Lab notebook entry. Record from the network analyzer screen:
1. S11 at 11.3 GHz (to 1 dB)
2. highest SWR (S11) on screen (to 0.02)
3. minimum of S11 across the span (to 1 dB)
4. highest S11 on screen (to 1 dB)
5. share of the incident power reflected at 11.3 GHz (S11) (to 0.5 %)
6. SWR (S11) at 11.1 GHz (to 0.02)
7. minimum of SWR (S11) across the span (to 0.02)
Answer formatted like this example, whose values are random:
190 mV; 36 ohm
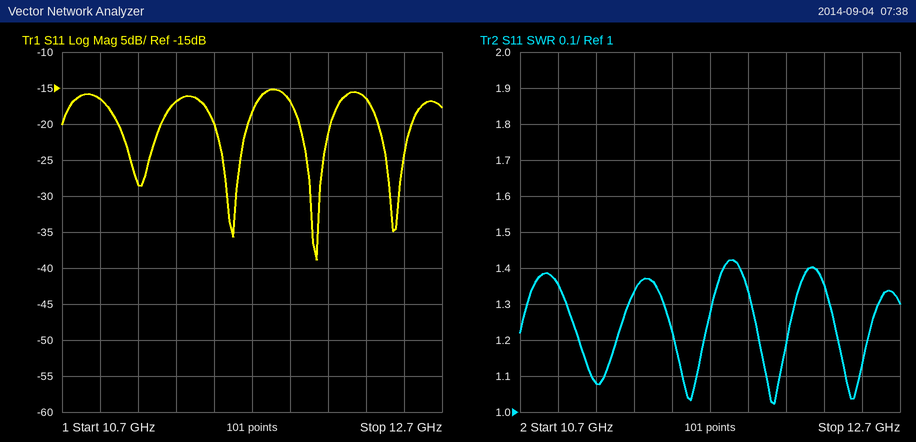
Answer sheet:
-17 dB; 1.42; -39 dB; -15 dB; 2.0 %; 1.08; 1.02
